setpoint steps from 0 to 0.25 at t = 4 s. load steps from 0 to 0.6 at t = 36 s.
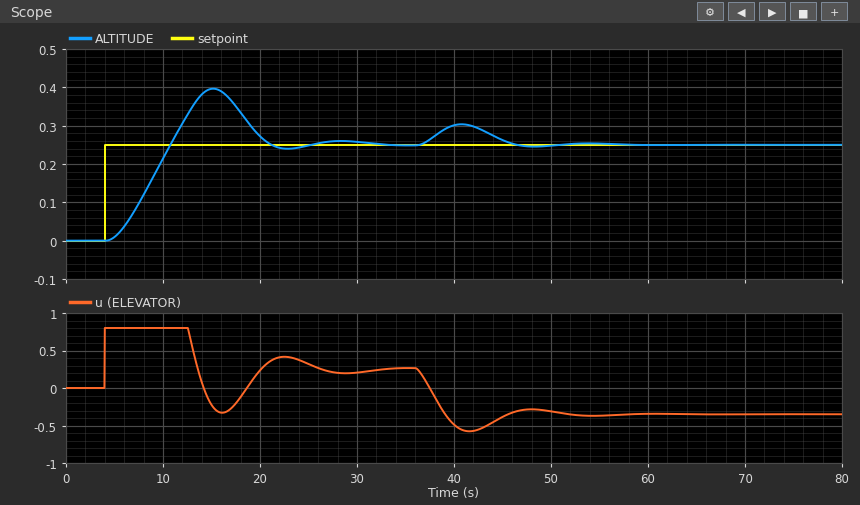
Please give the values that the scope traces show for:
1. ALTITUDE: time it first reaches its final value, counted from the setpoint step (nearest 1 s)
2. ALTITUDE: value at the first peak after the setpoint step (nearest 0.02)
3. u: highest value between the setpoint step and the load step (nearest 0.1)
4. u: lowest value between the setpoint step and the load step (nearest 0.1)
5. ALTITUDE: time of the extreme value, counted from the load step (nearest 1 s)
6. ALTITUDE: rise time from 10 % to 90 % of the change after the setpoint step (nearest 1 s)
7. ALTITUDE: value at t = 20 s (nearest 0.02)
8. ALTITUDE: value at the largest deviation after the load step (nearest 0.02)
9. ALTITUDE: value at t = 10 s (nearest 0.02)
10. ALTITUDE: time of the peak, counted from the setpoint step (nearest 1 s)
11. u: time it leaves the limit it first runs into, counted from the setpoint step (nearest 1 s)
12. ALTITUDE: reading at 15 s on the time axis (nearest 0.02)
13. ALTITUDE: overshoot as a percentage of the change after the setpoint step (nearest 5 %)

7 s
0.40
0.8
-0.3
5 s
5 s
0.28
0.30
0.22
11 s
9 s
0.40
60 %
